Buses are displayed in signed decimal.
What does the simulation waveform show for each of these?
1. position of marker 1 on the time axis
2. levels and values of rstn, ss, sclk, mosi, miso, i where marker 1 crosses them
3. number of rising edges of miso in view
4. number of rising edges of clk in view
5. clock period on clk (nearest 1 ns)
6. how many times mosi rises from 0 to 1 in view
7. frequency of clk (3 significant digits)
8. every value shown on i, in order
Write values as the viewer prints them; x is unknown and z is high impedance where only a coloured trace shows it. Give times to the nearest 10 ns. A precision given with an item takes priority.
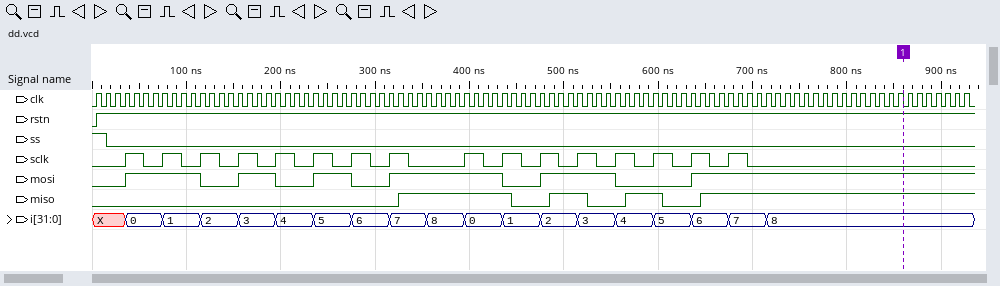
860 ns
rstn=1, ss=0, sclk=0, mosi=1, miso=1, i=8
4
93
10 ns
6
100 MHz
X, 0, 1, 2, 3, 4, 5, 6, 7, 8, 0, 1, 2, 3, 4, 5, 6, 7, 8
